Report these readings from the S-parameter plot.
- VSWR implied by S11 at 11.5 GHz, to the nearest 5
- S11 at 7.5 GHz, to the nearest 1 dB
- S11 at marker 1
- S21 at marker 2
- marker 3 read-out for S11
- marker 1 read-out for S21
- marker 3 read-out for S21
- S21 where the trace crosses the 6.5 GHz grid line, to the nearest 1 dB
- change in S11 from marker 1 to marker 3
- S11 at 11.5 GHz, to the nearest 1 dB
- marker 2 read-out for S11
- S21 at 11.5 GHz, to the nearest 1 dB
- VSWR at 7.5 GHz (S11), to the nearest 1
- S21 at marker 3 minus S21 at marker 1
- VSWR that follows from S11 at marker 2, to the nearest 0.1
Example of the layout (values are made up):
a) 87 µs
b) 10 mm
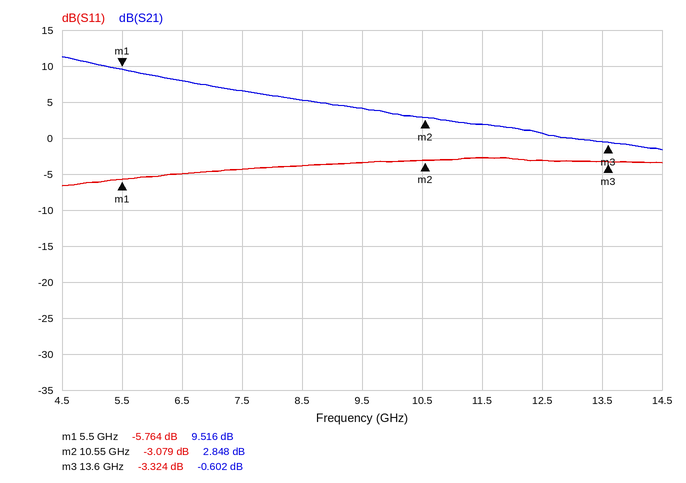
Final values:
a) 5
b) -4 dB
c) -5.764 dB
d) 2.848 dB
e) -3.324 dB
f) 9.516 dB
g) -0.602 dB
h) 8 dB
i) 2.440 dB
j) -3 dB
k) -3.079 dB
l) 2 dB
m) 4
n) -10.118 dB
o) 5.7
